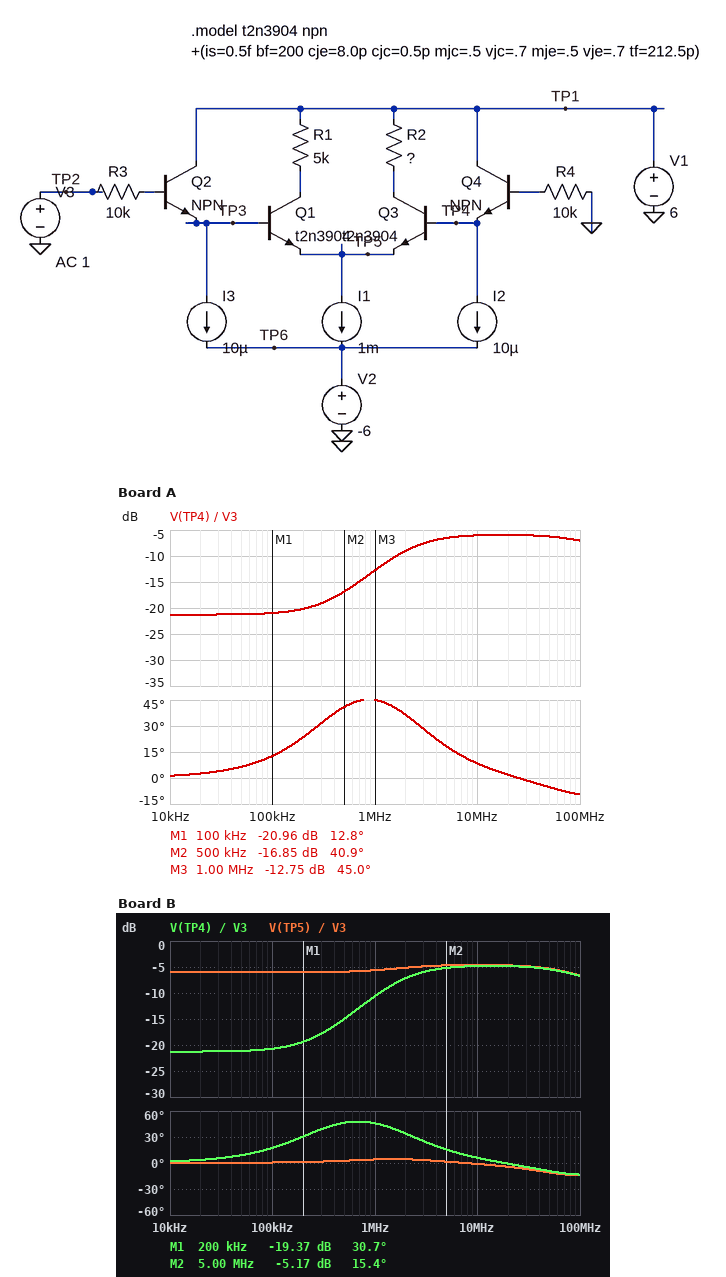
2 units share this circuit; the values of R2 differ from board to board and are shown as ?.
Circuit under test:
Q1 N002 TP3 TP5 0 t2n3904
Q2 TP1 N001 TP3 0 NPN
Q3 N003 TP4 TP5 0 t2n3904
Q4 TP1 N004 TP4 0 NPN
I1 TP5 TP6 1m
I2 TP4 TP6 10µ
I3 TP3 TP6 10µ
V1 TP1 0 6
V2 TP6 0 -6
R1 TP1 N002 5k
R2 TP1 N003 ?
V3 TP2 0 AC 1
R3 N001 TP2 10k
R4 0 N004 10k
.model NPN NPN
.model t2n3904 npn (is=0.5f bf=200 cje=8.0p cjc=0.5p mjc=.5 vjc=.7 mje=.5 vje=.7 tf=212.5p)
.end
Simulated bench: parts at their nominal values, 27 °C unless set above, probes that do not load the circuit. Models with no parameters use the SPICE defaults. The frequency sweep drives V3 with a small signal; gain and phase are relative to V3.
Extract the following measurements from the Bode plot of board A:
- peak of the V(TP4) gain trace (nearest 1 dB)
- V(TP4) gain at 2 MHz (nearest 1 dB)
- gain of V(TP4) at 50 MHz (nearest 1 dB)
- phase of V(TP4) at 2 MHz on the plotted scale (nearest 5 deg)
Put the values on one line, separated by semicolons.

-6 dB; -9 dB; -6 dB; 35 deg
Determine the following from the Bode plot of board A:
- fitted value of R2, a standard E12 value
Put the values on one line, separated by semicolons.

5.6 kΩ
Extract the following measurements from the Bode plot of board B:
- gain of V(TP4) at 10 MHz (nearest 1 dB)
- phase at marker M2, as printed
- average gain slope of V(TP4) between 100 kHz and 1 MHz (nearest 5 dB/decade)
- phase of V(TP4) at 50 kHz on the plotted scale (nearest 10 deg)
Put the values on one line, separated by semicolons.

-5 dB; 15.4 deg; 10 dB/decade; 10 deg
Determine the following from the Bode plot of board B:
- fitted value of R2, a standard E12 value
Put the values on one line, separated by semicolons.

8.2 kΩ
